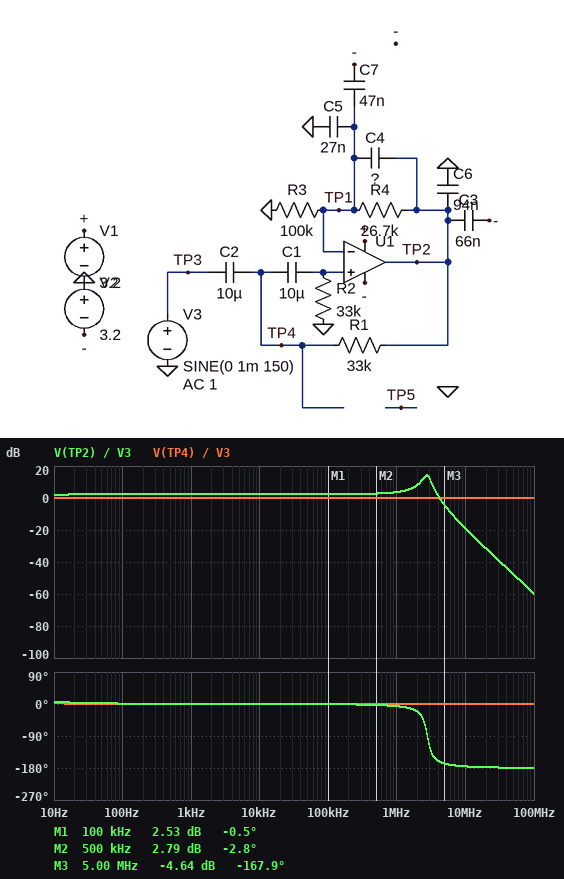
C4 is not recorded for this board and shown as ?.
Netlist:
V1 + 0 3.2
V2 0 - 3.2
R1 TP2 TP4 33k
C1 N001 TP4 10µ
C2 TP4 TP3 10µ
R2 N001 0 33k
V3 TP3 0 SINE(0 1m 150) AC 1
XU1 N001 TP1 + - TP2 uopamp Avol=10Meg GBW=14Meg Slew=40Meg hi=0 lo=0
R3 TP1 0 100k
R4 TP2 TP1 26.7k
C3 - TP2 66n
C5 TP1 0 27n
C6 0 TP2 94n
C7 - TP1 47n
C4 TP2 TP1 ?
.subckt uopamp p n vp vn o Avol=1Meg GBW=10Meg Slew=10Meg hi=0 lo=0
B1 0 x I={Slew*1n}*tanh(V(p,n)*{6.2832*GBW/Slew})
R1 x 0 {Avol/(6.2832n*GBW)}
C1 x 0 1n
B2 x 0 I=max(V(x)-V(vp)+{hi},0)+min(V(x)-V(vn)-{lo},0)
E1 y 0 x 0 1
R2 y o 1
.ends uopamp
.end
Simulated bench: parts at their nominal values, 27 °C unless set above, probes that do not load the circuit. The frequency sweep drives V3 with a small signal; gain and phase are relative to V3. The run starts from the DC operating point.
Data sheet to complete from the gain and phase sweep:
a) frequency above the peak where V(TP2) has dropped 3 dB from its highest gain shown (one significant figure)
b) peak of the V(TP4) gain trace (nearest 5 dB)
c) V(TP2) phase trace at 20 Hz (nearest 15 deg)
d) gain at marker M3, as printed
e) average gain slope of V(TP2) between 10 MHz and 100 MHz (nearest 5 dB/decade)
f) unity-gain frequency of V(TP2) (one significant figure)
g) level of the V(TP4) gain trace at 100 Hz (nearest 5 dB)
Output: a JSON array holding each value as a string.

["3 MHz", "0 dB", "0 deg", "-4.64 dB", "-40 dB/decade", "4 MHz", "0 dB"]
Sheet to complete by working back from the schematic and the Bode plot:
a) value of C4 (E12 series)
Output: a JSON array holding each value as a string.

["220 nF"]
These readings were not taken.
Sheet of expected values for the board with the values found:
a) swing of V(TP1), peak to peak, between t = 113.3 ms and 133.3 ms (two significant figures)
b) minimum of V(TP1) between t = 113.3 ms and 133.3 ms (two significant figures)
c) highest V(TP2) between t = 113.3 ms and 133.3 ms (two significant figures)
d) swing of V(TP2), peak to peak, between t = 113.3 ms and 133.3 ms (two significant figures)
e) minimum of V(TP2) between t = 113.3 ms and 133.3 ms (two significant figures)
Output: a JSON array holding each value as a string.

["2.0 mV", "-1.0 mV", "1.3 mV", "2.7 mV", "-1.3 mV"]
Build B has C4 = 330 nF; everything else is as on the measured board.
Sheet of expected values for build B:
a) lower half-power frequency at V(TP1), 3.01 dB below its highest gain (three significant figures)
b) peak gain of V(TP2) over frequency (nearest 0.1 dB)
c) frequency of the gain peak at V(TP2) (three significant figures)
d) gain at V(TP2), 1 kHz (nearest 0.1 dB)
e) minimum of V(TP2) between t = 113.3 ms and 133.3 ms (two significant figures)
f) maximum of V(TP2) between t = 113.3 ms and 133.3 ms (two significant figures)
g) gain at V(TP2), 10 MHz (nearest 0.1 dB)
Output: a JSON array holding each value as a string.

["2.44 MHz", "13.8 dB", "2.83 MHz", "1.8 dB", "-1.2 mV", "1.2 mV", "-19.2 dB"]
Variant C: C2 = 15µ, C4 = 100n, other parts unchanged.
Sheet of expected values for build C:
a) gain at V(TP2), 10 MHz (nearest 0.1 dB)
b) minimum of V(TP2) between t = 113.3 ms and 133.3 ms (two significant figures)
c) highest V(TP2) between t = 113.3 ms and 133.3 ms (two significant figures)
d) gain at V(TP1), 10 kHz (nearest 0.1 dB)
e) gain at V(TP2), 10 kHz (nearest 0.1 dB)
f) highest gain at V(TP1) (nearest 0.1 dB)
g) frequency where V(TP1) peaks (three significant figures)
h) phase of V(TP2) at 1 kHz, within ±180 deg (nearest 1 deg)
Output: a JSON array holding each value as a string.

["-18.6 dB", "-1.7 mV", "1.7 mV", "0 dB", "4.8 dB", "10.2 dB", "2.45 MHz", "1 deg"]
